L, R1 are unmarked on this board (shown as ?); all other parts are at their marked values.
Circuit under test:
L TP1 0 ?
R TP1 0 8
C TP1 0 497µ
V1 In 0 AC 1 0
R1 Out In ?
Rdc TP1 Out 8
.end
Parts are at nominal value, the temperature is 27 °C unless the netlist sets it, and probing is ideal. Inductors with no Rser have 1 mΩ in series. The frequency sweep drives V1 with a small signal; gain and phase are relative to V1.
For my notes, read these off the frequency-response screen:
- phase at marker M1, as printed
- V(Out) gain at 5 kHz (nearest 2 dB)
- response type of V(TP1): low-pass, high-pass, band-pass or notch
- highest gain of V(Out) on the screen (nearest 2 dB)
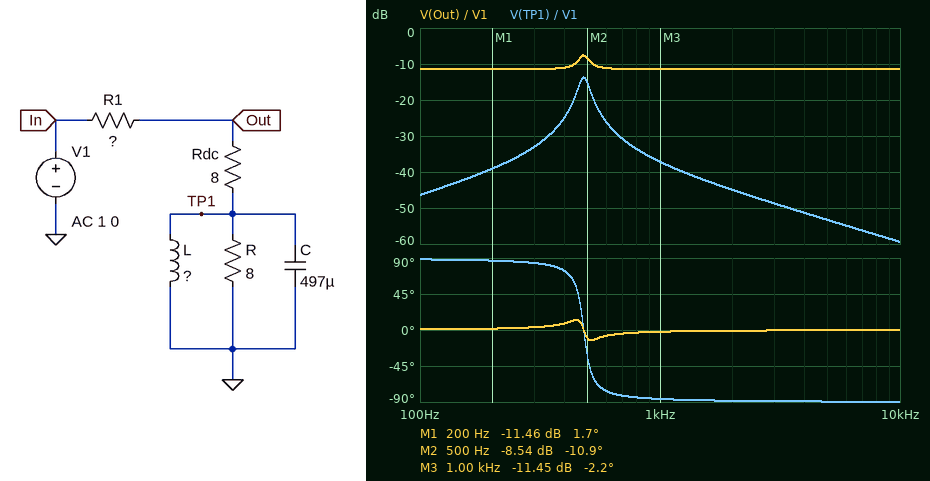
1.7 deg
-12 dB
band-pass
-8 dB
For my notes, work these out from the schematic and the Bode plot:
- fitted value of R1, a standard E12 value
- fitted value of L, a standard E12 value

22 Ω
220 µH
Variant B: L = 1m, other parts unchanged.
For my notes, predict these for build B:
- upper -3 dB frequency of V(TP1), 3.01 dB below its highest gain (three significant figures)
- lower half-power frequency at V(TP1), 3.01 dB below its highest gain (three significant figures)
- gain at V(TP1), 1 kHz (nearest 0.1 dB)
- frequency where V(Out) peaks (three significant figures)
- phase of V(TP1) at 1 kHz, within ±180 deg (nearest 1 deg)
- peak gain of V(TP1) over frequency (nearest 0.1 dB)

253 Hz
202 Hz
-39.0 dB
226 Hz
-87 deg
-13.6 dB
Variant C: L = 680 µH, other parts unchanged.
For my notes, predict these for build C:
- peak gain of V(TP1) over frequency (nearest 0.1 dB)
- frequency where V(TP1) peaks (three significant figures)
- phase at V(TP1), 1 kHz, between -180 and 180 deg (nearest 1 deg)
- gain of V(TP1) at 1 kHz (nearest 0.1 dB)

-13.6 dB
274 Hz
-87 deg
-38.8 dB
